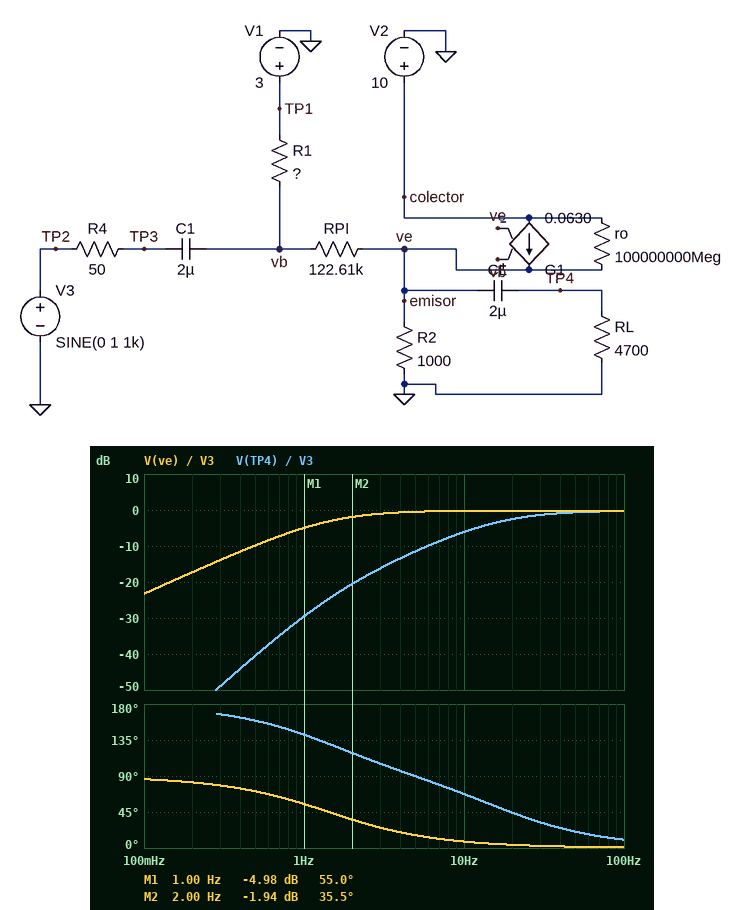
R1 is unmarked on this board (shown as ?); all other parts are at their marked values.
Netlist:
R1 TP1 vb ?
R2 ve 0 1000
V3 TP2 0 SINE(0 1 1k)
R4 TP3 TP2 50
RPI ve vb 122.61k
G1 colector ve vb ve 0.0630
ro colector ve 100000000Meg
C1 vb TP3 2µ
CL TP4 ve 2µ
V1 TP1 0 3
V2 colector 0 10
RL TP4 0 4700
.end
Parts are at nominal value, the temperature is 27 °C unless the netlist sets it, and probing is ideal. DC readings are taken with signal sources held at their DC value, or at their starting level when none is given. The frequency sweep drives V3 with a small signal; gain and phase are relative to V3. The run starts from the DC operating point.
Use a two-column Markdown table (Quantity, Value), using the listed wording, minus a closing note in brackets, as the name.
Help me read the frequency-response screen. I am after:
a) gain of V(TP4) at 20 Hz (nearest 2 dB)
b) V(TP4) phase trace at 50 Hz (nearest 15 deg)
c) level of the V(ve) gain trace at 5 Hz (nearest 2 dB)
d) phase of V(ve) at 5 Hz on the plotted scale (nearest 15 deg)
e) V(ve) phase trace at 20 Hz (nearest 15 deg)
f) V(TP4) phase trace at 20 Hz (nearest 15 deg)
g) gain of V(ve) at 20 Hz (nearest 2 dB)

| Quantity | Value |
|---|---|
| gain of V(TP4) at 20 Hz | -2 dB |
| V(TP4) phase trace at 50 Hz | 15 deg |
| level of the V(ve) gain trace at 5 Hz | 0 dB |
| phase of V(ve) at 5 Hz on the plotted scale | 15 deg |
| V(ve) phase trace at 20 Hz | 0 deg |
| V(TP4) phase trace at 20 Hz | 45 deg |
| gain of V(ve) at 20 Hz | 0 dB |
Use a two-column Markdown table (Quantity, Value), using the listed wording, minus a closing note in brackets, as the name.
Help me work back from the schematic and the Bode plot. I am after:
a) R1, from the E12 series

| Quantity | Value |
|---|---|
| R1, from the E12 series | 56 kΩ |
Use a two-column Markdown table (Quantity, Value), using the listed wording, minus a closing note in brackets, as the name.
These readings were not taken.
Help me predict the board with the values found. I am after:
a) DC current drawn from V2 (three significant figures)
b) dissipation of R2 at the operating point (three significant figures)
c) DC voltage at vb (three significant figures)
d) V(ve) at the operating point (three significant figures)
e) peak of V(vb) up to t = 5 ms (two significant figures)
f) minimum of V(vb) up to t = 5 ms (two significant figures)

| Quantity | Value |
|---|---|
| DC current drawn from V2 | 2.93 mA |
| dissipation of R2 at the operating point | 8.60 mW |
| DC voltage at vb | 2.98 V |
| V(ve) at the operating point | 2.93 V |
| peak of V(vb) up to t = 5 ms | 4.0 V |
| minimum of V(vb) up to t = 5 ms | 2.0 V |
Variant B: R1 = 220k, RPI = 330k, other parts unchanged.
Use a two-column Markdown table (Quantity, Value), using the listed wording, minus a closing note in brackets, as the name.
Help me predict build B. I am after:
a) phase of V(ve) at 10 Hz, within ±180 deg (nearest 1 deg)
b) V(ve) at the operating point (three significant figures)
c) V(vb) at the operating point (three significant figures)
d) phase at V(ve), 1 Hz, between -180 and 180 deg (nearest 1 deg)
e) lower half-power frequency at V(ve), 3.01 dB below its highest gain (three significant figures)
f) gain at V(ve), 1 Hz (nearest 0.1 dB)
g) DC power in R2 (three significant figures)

| Quantity | Value |
|---|---|
| phase of V(ve) at 10 Hz, within ±180 deg | 2 deg |
| V(ve) at the operating point | 2.92 V |
| V(vb) at the operating point | 2.97 V |
| phase at V(ve), 1 Hz, between -180 and 180 deg | 20 deg |
| lower half-power frequency at V(ve), 3.01 dB below its highest gain | 364 mHz |
| gain at V(ve), 1 Hz | -0.7 dB |
| DC power in R2 | 8.54 mW |
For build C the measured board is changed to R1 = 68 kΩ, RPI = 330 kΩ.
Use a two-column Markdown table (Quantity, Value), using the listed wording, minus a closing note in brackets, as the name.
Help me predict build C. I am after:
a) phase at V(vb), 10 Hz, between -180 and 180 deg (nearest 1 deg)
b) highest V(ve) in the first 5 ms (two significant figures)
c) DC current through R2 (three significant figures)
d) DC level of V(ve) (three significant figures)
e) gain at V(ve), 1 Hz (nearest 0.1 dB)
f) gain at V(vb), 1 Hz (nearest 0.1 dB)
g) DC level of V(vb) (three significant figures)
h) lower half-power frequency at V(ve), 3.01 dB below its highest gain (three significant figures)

| Quantity | Value |
|---|---|
| phase at V(vb), 10 Hz, between -180 and 180 deg | 7 deg |
| highest V(ve) in the first 5 ms | 3.9 V |
| DC current through R2 | 2.94 mA |
| DC level of V(ve) | 2.94 V |
| gain at V(ve), 1 Hz | -3.9 dB |
| gain at V(vb), 1 Hz | -3.8 dB |
| DC level of V(vb) | 2.99 V |
| lower half-power frequency at V(ve), 3.01 dB below its highest gain | 1.17 Hz |
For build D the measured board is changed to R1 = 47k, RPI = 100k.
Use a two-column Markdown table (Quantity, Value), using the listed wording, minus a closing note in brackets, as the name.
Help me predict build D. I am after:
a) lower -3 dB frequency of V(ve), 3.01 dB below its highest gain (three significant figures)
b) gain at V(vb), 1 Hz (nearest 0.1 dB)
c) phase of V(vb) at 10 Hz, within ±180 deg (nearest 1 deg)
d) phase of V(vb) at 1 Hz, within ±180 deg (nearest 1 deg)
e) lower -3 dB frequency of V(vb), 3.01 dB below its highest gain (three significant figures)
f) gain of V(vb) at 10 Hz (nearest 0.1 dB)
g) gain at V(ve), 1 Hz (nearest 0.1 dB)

| Quantity | Value |
|---|---|
| lower -3 dB frequency of V(ve), 3.01 dB below its highest gain | 1.69 Hz |
| gain at V(vb), 1 Hz | -5.9 dB |
| phase of V(vb) at 10 Hz, within ±180 deg | 10 deg |
| phase of V(vb) at 1 Hz, within ±180 deg | 60 deg |
| lower -3 dB frequency of V(vb), 3.01 dB below its highest gain | 1.70 Hz |
| gain of V(vb) at 10 Hz | -0.1 dB |
| gain at V(ve), 1 Hz | -6.1 dB |
